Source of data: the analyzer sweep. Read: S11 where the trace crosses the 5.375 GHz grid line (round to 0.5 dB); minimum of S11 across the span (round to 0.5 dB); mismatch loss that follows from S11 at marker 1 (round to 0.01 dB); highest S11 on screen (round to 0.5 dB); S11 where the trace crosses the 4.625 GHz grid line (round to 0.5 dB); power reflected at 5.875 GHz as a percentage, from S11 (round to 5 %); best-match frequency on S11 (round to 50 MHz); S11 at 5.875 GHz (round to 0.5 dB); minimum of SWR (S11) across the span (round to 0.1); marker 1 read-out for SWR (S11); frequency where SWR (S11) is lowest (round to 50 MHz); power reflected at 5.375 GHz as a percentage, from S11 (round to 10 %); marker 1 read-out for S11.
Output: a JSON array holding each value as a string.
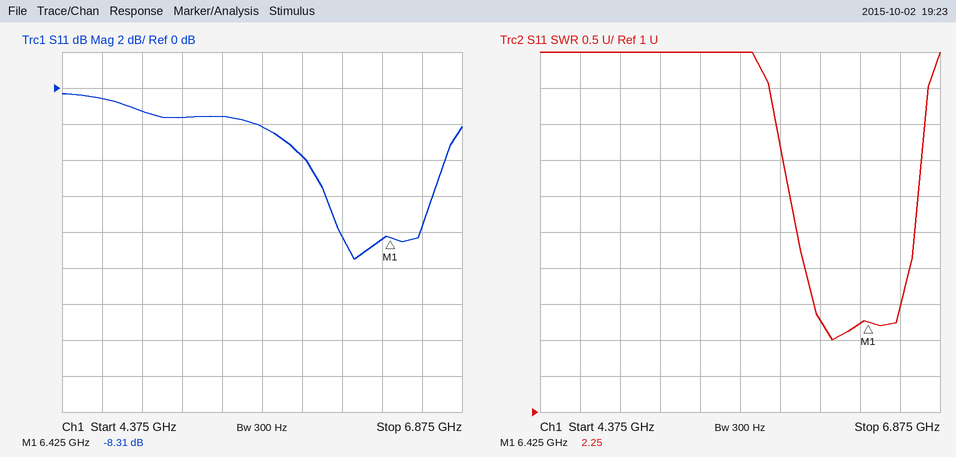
["-1.5 dB", "-9.5 dB", "0.69 dB", "-0.5 dB", "-0.5 dB", "40 %", "6.20 GHz", "-4.0 dB", "2.0", "2.25", "6.20 GHz", "70 %", "-8.31 dB"]
